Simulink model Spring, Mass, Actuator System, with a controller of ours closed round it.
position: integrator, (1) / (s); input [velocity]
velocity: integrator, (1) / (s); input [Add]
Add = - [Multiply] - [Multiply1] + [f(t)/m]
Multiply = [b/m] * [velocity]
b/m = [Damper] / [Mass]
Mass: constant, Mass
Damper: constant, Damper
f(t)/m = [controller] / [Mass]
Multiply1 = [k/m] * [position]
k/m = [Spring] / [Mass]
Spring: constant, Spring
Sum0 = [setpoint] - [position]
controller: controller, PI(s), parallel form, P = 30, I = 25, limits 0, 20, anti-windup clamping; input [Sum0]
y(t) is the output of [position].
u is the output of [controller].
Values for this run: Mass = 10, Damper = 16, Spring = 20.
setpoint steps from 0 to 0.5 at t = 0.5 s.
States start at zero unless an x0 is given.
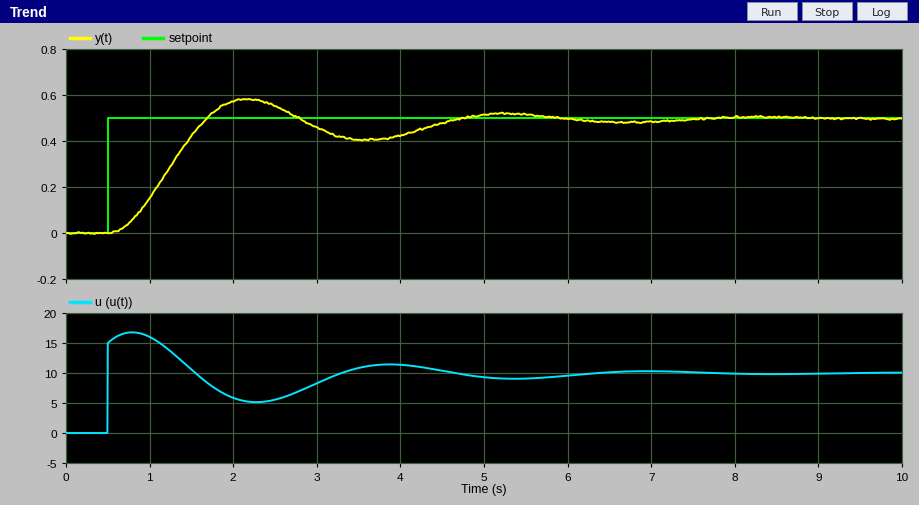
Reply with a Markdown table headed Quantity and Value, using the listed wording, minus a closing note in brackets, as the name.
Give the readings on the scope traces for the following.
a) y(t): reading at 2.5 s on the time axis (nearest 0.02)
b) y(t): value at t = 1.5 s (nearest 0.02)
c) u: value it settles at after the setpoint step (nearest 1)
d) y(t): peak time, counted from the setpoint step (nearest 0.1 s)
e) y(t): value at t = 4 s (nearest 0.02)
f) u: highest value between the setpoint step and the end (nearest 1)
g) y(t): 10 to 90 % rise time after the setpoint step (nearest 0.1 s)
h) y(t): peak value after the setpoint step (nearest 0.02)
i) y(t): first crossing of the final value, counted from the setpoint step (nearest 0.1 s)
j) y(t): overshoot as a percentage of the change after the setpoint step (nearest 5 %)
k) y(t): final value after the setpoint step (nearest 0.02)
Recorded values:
| Quantity | Value |
|---|---|
| y(t): reading at 2.5 s on the time axis | 0.56 |
| y(t): value at t = 1.5 s | 0.42 |
| u: value it settles at after the setpoint step | 10 |
| y(t): peak time, counted from the setpoint step | 1.7 s |
| y(t): value at t = 4 s | 0.42 |
| u: highest value between the setpoint step and the end | 17 |
| y(t): 10 to 90 % rise time after the setpoint step | 0.8 s |
| y(t): peak value after the setpoint step | 0.58 |
| y(t): first crossing of the final value, counted from the setpoint step | 1.2 s |
| y(t): overshoot as a percentage of the change after the setpoint step | 15 % |
| y(t): final value after the setpoint step | 0.50 |
